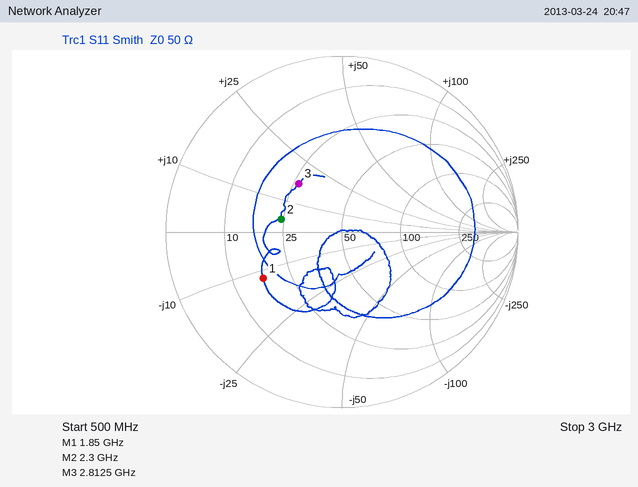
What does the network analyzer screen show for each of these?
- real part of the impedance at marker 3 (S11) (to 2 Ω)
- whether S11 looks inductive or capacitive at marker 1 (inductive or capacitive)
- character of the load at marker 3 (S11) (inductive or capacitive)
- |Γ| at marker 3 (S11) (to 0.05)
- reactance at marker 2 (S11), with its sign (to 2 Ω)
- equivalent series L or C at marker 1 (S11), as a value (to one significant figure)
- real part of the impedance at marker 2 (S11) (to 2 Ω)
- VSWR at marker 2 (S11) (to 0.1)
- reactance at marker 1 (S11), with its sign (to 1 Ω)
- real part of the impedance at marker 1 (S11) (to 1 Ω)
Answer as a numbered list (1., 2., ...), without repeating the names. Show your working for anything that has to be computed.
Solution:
1. 26 Ω
2. capacitive
3. inductive
4. 0.35
5. +4 Ω
6. C = 1/(2π × 1.85 GHz × 12 Ω) ≈ 7 pF
7. 24 Ω
8. 2.1
9. -12 Ω
10. 17 Ω
